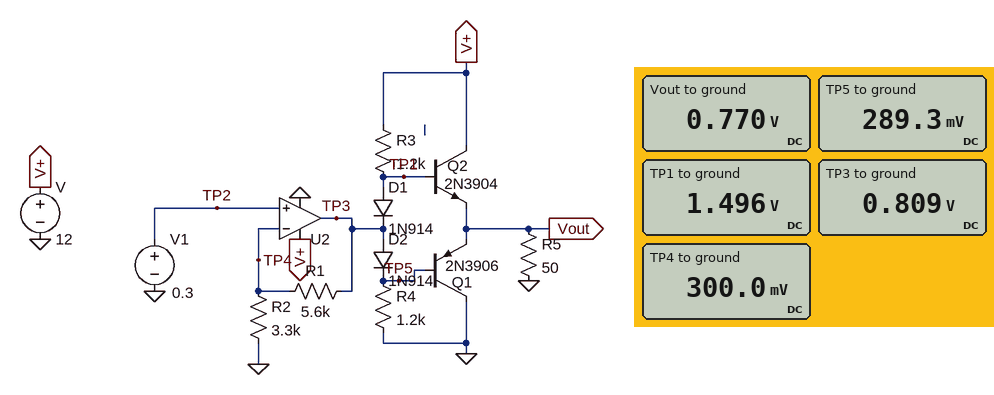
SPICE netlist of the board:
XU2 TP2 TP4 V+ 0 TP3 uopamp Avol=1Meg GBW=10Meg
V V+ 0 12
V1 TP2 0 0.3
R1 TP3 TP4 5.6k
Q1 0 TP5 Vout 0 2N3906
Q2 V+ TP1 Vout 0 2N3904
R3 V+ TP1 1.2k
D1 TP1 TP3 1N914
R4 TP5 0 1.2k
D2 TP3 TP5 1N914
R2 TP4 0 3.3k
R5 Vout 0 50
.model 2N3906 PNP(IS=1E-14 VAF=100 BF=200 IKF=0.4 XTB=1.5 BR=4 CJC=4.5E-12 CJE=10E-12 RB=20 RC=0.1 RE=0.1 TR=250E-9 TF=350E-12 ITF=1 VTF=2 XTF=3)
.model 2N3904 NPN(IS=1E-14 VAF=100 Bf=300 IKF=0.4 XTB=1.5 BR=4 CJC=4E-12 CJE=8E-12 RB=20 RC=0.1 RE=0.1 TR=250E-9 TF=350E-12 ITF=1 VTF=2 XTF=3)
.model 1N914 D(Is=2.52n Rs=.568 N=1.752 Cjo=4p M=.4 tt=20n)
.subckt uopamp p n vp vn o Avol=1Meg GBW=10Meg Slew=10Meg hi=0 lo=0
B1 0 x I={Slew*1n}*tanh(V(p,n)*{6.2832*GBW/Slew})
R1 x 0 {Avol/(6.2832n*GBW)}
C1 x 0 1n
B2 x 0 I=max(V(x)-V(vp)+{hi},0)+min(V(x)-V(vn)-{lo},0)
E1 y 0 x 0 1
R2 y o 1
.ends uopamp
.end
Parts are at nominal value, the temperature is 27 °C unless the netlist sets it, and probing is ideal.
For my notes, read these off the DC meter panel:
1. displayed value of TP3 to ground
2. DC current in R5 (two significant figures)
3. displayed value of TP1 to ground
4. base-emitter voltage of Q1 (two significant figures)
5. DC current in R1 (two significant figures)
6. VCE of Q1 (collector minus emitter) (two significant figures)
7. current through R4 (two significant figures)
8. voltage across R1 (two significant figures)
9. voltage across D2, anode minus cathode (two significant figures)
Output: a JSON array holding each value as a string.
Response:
["0.809 V", "15 mA", "1.496 V", "-480 mV", "91 µA", "-770 mV", "240 µA", "510 mV", "520 mV"]
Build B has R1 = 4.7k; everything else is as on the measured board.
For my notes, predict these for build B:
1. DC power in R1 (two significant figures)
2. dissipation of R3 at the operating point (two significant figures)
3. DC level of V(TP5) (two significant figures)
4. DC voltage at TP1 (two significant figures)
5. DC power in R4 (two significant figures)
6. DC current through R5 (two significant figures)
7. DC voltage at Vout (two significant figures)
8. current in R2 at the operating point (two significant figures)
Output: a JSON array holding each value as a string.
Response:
["39 µW", "93 mW", "220 mV", "1.4 V", "40 µW", "14 mA", "690 mV", "91 µA"]
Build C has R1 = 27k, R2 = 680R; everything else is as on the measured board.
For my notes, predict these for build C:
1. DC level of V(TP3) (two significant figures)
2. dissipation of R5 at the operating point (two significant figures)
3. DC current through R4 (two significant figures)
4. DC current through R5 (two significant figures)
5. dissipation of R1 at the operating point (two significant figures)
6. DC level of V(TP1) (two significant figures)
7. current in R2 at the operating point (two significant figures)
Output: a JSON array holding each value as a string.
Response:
["12 V", "2.0 W", "9.4 mA", "200 mA", "5.1 mW", "11 V", "430 µA"]
